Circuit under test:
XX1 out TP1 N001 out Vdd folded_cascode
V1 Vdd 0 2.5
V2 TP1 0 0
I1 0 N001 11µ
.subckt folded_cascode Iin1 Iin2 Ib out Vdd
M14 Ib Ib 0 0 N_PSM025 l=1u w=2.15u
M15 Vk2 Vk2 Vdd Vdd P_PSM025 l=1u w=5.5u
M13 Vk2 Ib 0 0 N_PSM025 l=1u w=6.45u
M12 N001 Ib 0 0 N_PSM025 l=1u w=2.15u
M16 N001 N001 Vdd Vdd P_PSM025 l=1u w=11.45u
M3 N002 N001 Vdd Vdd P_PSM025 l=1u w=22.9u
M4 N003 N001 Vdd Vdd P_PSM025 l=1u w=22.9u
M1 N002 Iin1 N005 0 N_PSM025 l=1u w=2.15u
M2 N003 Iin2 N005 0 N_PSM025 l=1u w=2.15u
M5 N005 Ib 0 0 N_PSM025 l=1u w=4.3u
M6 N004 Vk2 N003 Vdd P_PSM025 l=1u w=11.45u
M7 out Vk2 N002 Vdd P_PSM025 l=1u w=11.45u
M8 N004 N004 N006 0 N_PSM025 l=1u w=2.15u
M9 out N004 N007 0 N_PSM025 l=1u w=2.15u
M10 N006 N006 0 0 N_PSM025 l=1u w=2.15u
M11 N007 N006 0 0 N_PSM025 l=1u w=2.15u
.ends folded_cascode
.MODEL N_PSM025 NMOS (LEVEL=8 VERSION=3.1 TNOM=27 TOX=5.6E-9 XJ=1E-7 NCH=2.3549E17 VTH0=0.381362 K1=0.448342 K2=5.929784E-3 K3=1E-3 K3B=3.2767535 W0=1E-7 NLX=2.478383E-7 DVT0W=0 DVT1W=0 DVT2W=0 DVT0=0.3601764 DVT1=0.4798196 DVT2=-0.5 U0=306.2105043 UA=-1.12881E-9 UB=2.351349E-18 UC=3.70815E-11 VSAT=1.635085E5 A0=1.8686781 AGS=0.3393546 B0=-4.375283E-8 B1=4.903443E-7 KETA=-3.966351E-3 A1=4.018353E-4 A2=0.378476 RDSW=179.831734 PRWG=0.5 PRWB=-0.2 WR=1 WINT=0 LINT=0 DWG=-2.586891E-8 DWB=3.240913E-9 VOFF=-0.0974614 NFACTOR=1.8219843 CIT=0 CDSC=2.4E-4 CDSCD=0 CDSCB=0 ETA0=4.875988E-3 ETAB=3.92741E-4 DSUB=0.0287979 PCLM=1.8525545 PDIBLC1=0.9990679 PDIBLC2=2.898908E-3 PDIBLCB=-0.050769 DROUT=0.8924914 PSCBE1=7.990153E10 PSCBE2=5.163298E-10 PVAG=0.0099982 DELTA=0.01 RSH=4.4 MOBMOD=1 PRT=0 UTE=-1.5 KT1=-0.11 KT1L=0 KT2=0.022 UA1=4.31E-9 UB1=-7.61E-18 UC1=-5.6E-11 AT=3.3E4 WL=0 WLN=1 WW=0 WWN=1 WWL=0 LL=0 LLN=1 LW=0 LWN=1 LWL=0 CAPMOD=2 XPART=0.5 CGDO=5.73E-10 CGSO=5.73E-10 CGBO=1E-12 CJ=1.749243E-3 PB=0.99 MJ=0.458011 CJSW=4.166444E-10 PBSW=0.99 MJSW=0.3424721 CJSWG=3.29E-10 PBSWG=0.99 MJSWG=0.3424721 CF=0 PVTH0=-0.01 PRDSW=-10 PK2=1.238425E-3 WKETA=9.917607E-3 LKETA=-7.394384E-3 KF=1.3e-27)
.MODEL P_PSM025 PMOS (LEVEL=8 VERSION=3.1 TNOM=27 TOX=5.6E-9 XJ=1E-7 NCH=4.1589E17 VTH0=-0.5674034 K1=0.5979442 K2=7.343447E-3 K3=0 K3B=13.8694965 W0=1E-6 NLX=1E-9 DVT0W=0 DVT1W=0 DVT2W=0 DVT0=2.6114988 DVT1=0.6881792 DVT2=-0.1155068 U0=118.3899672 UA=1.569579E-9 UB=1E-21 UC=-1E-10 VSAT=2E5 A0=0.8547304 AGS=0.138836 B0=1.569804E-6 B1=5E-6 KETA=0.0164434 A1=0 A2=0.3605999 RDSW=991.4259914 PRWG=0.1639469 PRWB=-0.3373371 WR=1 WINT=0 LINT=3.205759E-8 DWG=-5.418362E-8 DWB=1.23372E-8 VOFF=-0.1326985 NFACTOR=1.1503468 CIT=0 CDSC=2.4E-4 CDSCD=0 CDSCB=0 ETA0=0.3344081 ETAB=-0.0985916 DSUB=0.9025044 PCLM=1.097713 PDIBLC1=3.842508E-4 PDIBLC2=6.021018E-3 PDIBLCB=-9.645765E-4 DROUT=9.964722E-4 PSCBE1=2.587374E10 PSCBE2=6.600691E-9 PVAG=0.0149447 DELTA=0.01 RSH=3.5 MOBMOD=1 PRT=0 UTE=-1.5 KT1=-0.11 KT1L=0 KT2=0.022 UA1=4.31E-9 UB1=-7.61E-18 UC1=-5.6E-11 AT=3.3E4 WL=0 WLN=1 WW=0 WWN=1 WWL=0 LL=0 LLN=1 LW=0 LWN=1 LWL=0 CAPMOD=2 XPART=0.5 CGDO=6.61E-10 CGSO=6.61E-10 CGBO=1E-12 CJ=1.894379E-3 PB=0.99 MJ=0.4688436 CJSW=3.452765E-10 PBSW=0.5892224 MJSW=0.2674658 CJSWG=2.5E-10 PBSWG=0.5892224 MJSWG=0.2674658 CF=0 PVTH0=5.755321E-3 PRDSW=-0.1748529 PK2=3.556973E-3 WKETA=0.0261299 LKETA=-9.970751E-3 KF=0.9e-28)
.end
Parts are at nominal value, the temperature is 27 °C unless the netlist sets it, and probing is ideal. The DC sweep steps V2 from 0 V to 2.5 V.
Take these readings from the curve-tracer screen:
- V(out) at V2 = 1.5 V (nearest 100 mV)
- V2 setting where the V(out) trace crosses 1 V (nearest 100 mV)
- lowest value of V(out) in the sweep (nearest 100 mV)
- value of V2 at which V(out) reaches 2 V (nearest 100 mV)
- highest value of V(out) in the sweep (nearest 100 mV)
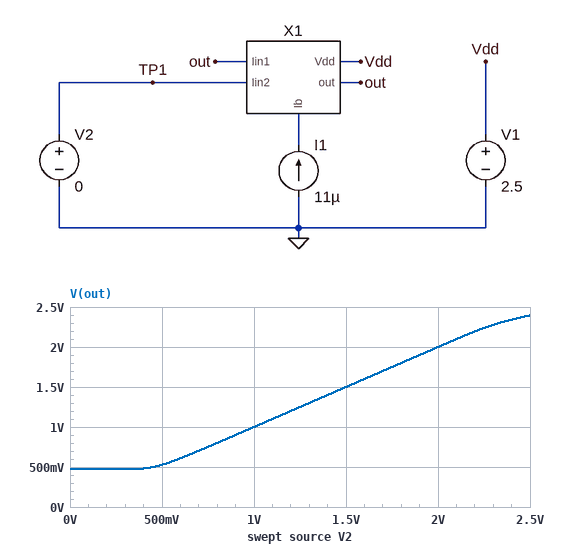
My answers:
1.5 V
1.0 V
500 mV
2.0 V
2.4 V
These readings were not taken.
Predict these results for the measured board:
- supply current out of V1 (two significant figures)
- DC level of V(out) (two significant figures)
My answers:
91 µA
470 mV
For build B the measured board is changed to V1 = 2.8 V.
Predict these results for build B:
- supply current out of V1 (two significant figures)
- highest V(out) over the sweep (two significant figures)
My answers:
94 µA
2.5 V
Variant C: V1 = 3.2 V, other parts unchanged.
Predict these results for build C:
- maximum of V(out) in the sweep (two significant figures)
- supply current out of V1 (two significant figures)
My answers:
2.5 V
97 µA
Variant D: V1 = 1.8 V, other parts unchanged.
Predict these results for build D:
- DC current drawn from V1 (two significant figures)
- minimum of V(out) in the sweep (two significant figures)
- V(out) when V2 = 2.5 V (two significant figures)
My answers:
83 µA
570 mV
1.8 V
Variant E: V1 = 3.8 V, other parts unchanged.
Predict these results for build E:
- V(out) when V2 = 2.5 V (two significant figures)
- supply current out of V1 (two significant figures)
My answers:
2.5 V
100 µA
